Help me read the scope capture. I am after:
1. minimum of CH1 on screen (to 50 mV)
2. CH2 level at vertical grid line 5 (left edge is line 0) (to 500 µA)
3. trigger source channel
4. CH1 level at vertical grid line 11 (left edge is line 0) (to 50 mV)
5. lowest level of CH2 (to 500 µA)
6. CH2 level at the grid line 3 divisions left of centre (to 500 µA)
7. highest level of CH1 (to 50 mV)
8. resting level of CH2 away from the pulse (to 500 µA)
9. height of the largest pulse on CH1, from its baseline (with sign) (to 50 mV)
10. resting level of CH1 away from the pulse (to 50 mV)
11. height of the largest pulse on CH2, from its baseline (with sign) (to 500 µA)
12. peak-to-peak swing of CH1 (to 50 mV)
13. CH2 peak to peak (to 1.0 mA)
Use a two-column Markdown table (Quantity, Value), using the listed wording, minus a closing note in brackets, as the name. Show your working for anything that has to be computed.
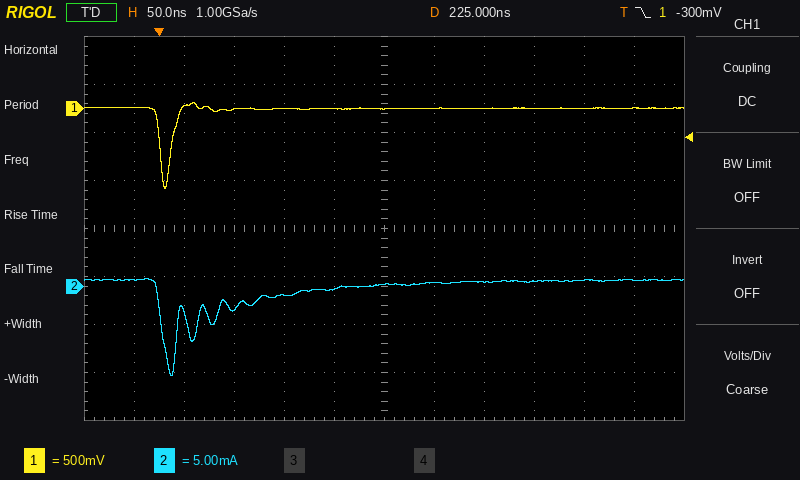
| Quantity | Value |
|---|---|
| minimum of CH1 on screen | -850 mV |
| CH2 level at vertical grid line 5 (left edge is line 0) | -500 µA |
| trigger source channel | CH1 |
| CH1 level at vertical grid line 11 (left edge is line 0) | 0 mV |
| lowest level of CH2 | -9.5 mA |
| CH2 level at the grid line 3 divisions left of centre | -2.5 mA |
| highest level of CH1 | 50 mV |
| resting level of CH2 away from the pulse | 500 µA |
| height of the largest pulse on CH1, from its baseline (with sign) | -850 mV − (0 mV) = -850 mV |
| resting level of CH1 away from the pulse | 0 mV |
| height of the largest pulse on CH2, from its baseline (with sign) | -9.5 mA − (500 µA) = -10.0 mA |
| peak-to-peak swing of CH1 | 50 mV − (-850 mV) = 900 mV |
| CH2 peak to peak | 10.0 mA |
